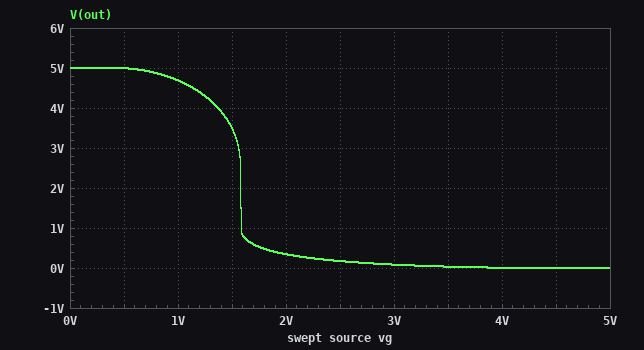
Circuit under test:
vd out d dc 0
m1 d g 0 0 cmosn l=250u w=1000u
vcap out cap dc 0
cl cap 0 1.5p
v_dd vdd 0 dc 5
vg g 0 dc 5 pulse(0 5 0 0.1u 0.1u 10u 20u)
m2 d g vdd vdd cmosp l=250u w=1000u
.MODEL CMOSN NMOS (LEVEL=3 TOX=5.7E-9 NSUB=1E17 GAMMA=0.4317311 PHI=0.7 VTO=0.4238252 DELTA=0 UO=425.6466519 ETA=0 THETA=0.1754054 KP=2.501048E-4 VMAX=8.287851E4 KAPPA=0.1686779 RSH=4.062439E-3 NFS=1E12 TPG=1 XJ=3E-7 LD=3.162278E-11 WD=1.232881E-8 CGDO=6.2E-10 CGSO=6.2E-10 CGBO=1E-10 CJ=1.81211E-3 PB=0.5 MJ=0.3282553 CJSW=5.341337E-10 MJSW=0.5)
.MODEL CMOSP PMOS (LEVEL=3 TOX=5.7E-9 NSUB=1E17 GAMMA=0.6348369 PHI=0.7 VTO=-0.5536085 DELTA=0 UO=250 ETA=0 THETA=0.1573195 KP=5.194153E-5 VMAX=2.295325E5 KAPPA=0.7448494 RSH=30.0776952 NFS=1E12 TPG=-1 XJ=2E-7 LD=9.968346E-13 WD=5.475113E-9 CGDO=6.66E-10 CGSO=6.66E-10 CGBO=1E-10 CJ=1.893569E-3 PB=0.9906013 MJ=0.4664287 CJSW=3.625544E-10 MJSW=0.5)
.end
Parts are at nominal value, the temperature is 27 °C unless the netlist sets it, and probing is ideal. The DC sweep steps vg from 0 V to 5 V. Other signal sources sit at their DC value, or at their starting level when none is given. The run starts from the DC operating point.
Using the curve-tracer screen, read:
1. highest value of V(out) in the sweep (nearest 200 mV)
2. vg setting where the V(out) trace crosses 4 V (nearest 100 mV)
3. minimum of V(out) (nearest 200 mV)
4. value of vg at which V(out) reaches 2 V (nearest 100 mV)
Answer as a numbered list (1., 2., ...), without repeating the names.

1. 5.0 V
2. 1.4 V
3. 0 V
4. 1.6 V
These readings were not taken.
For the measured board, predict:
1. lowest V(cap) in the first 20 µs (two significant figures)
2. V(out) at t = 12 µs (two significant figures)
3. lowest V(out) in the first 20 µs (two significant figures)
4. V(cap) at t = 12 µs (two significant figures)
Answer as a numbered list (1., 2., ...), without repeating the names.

1. -760 mV
2. 3.8 V
3. -760 mV
4. 3.8 V
